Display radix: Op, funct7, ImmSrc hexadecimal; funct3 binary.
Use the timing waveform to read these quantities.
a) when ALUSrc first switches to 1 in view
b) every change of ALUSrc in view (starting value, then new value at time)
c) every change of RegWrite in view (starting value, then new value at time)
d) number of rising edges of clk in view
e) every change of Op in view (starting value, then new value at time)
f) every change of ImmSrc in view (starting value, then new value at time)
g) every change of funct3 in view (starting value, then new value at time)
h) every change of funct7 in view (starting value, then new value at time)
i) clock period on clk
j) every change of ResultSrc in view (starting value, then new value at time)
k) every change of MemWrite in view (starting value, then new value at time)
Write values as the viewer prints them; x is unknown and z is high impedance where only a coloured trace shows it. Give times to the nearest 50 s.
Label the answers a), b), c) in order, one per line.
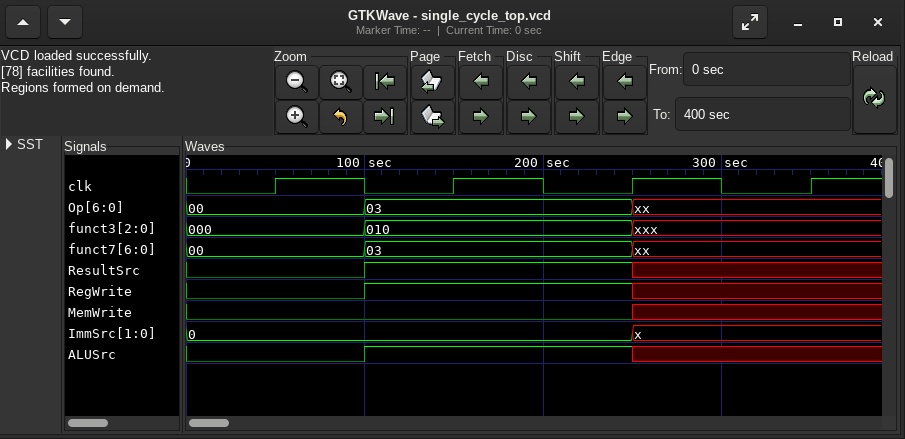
a) 100 s
b) 0, 1 at 100 s, x at 250 s
c) 0, 1 at 100 s, x at 250 s
d) 4
e) 00, 03 at 100 s, xx at 250 s
f) 0, x at 250 s
g) 000, 010 at 100 s, xxx at 250 s
h) 00, 03 at 100 s, xx at 250 s
i) 100 s
j) 0, 1 at 100 s, x at 250 s
k) 0, x at 250 s
